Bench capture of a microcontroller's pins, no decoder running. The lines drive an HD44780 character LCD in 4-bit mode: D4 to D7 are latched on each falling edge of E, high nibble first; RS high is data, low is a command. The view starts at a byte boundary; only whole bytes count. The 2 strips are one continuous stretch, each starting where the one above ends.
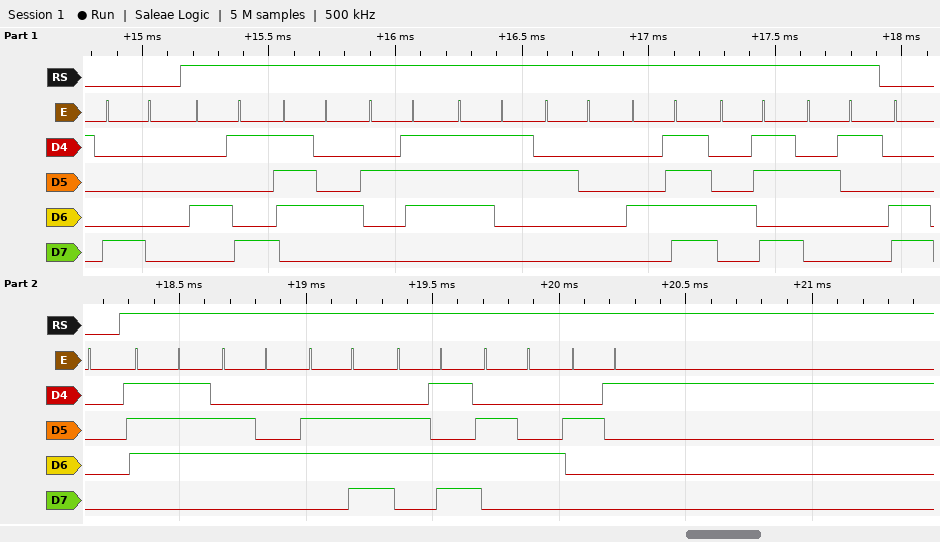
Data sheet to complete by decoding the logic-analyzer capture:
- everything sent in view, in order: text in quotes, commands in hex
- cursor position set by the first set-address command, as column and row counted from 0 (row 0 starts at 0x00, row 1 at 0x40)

0x80 "It's OK!" 0xC0 "wdnmd!"
column 0, row 0
